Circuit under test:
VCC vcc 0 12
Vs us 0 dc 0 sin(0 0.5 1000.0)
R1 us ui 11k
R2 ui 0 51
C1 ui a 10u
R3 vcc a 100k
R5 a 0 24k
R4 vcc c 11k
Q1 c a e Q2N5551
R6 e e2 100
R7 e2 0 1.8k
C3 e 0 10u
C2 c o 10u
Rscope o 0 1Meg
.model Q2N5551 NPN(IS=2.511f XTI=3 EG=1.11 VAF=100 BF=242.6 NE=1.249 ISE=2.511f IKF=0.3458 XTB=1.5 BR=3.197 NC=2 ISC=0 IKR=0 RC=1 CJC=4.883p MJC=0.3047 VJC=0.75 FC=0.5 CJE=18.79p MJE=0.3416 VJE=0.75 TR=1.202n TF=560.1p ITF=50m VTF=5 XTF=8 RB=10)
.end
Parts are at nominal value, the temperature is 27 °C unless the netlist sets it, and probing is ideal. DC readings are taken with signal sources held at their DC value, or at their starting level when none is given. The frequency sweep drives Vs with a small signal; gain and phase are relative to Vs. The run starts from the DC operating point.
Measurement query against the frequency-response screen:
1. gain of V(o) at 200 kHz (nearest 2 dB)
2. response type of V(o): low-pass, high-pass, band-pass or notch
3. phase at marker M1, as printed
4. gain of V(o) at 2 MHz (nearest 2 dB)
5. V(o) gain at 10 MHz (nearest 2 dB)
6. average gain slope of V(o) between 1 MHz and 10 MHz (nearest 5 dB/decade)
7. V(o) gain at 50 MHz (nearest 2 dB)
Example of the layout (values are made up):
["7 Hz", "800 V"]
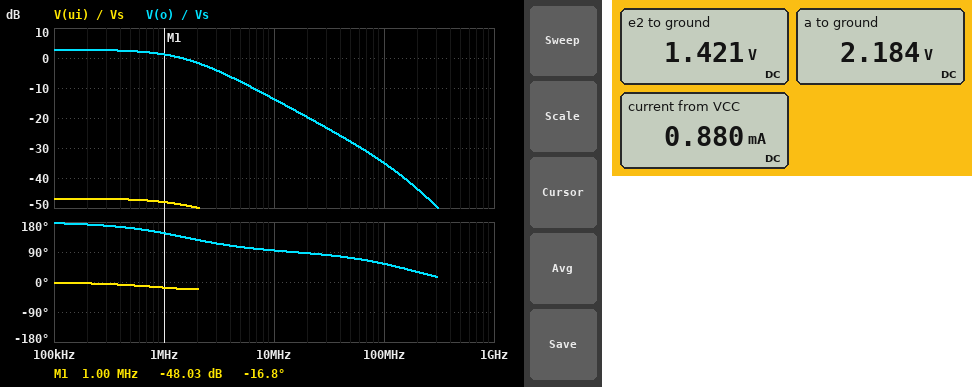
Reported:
["2 dB", "low-pass", "-16.8 deg", "-2 dB", "-14 dB", "-15 dB/decade", "-28 dB"]
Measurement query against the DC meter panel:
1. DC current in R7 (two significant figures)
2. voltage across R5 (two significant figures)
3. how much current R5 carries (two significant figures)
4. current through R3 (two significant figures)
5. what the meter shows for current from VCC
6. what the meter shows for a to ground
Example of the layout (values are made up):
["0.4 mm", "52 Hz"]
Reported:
["790 µA", "2.2 V", "91 µA", "98 µA", "0.880 mA", "2.184 V"]
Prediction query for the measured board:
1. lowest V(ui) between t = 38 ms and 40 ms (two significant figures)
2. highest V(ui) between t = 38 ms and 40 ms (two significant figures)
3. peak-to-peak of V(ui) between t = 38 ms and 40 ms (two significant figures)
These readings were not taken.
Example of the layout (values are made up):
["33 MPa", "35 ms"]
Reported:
["-2.3 mV", "2.3 mV", "4.6 mV"]
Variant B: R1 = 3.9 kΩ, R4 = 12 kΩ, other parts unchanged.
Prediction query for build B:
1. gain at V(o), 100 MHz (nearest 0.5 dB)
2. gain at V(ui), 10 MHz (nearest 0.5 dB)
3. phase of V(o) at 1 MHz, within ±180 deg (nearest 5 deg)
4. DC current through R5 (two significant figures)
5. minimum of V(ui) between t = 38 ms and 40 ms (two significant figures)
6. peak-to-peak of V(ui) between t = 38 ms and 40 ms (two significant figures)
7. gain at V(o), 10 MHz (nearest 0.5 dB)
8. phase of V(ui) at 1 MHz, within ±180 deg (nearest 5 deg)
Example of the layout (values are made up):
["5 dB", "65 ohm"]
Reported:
["-27.5 dB", "-44.5 dB", "140 deg", "91 µA", "-6.3 mV", "12 mV", "-6.0 dB", "-20 deg"]
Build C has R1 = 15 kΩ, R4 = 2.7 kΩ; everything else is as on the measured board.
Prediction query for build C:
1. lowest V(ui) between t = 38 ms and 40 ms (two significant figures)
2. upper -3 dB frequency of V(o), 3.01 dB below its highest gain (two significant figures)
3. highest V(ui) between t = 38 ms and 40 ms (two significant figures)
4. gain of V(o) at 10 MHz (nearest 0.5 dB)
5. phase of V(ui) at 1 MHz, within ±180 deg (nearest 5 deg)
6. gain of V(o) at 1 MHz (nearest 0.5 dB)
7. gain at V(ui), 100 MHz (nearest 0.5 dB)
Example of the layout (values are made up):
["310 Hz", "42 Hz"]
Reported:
["-1.7 mV", "8.2 MHz", "1.7 mV", "-15.5 dB", "-5 deg", "-11.5 dB", "-58.0 dB"]
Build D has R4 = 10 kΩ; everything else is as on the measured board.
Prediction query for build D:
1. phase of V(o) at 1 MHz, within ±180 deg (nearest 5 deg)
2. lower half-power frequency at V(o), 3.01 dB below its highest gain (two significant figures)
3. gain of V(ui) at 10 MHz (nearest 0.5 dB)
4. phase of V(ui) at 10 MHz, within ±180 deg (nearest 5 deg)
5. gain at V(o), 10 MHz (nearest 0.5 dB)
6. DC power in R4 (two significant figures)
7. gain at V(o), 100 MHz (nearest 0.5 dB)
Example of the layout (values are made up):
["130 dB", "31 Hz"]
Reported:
["150 deg", "460 Hz", "-53.0 dB", "-15 deg", "-13.0 dB", "6.1 mW", "-34.0 dB"]
